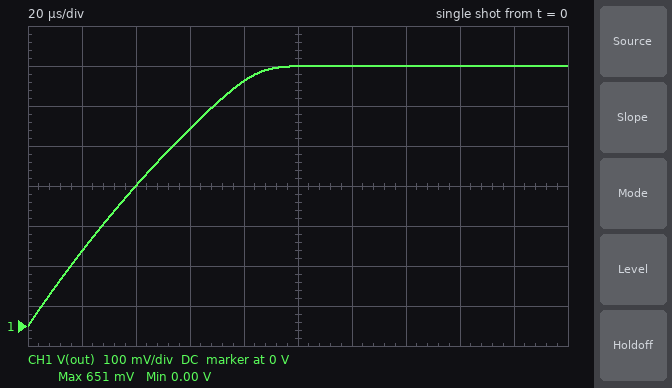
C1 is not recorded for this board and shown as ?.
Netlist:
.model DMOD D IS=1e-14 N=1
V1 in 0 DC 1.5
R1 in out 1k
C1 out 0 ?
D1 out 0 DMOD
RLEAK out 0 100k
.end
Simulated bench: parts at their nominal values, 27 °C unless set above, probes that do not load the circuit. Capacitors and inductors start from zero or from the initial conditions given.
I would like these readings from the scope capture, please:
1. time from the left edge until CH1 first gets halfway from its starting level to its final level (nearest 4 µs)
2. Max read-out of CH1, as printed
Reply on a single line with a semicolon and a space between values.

36 µs; 651 mV
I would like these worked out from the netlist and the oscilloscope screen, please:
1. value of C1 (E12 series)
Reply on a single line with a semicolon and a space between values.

150 nF
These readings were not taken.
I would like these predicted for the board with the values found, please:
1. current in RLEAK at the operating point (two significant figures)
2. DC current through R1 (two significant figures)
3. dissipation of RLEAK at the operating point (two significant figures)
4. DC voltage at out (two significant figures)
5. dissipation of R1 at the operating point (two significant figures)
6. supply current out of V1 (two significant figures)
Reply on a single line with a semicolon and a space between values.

6.5 µA; 850 µA; 4.2 µW; 650 mV; 720 µW; 850 µA
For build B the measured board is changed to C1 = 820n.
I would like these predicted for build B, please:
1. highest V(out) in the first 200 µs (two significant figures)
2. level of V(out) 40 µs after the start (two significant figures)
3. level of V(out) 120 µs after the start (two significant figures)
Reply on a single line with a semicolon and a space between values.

320 mV; 71 mV; 200 mV
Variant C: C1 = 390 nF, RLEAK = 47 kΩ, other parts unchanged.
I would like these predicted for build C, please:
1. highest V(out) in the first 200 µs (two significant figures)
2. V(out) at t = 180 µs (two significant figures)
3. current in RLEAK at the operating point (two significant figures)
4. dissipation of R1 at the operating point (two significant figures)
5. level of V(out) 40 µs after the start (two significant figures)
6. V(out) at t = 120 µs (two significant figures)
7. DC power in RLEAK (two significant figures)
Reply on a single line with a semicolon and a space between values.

600 mV; 550 mV; 14 µA; 720 µW; 150 mV; 400 mV; 9.0 µW
